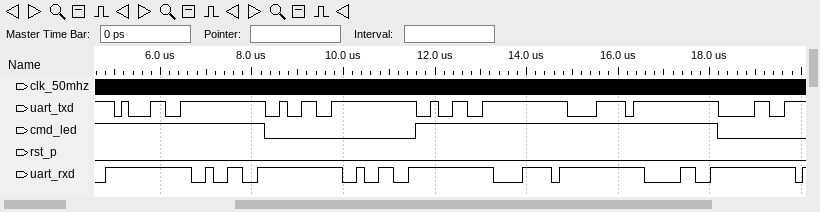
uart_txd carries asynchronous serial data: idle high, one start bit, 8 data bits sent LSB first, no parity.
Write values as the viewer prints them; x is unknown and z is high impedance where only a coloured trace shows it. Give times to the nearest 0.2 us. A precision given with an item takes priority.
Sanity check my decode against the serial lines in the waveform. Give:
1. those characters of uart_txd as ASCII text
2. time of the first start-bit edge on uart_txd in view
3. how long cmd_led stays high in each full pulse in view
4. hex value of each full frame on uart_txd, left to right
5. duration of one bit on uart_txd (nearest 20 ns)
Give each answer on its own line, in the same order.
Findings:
"122x0"
5 us
6.6 us
31, 32, 32, 78, 30
160 ns
